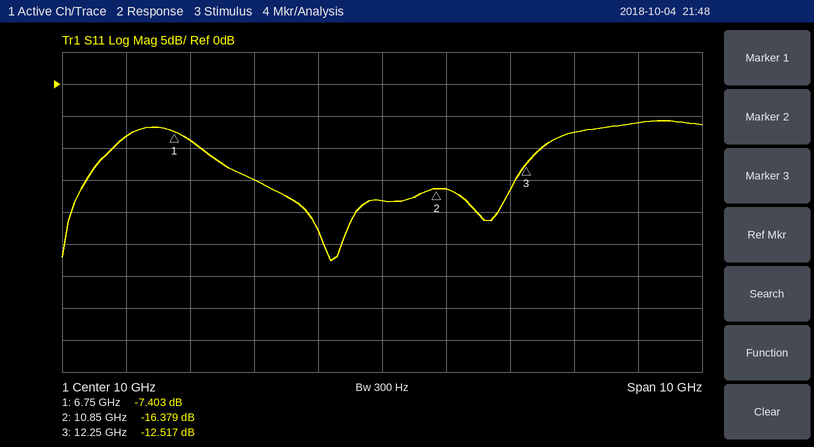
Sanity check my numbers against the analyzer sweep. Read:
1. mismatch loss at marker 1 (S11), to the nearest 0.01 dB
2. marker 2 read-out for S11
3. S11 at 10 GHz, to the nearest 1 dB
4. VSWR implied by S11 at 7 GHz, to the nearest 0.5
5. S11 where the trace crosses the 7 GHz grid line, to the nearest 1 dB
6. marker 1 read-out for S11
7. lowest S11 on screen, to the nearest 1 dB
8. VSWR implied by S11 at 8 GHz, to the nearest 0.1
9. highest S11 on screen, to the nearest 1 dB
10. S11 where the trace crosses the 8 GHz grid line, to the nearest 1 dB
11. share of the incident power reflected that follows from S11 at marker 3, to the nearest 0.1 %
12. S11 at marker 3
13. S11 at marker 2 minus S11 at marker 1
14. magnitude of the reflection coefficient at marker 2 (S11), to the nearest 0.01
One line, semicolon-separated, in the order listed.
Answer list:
0.87 dB; -16.379 dB; -18 dB; 2.0; -9 dB; -7.403 dB; -28 dB; 1.4; -6 dB; -15 dB; 5.6 %; -12.517 dB; -8.976 dB; 0.15
